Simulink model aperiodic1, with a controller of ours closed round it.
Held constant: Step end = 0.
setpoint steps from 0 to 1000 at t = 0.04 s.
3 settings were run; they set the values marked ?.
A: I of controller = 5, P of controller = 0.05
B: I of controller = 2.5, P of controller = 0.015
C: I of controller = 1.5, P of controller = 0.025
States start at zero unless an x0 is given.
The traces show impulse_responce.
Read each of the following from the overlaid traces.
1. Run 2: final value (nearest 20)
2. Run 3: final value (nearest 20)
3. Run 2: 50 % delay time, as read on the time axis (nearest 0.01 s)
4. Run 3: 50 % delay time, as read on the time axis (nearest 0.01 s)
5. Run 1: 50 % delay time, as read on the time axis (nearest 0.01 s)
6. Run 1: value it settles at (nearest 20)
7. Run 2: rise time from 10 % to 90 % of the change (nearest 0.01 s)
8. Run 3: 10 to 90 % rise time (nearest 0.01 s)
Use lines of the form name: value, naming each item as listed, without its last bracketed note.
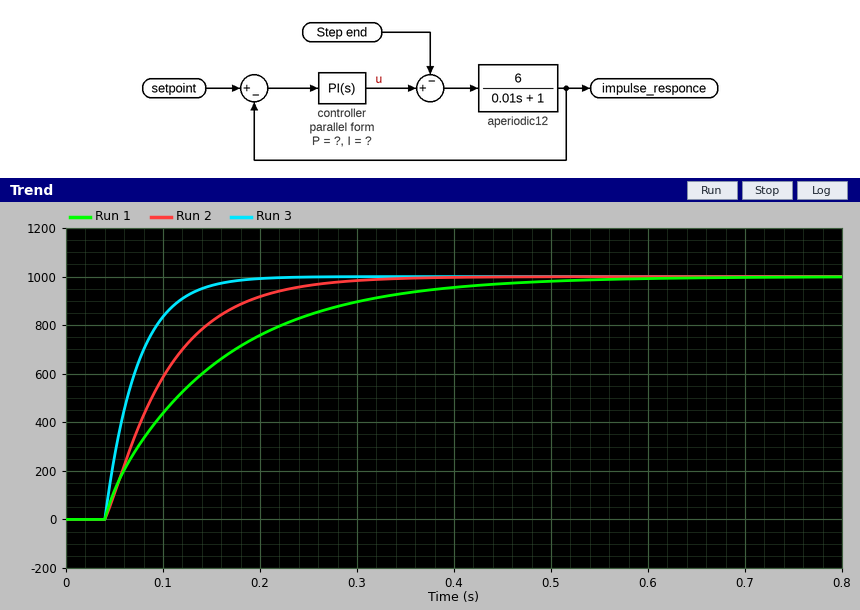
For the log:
Run 2: final value: 1000
Run 3: final value: 1000
Run 2: 50 % delay time, as read on the time axis: 0.09 s
Run 3: 50 % delay time, as read on the time axis: 0.06 s
Run 1: 50 % delay time, as read on the time axis: 0.11 s
Run 1: value it settles at: 1000
Run 2: rise time from 10 % to 90 % of the change: 0.14 s
Run 3: 10 to 90 % rise time: 0.07 s
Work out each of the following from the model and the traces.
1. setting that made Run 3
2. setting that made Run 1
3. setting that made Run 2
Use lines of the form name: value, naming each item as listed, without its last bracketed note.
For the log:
setting that made Run 3: A
setting that made Run 1: C
setting that made Run 2: B
